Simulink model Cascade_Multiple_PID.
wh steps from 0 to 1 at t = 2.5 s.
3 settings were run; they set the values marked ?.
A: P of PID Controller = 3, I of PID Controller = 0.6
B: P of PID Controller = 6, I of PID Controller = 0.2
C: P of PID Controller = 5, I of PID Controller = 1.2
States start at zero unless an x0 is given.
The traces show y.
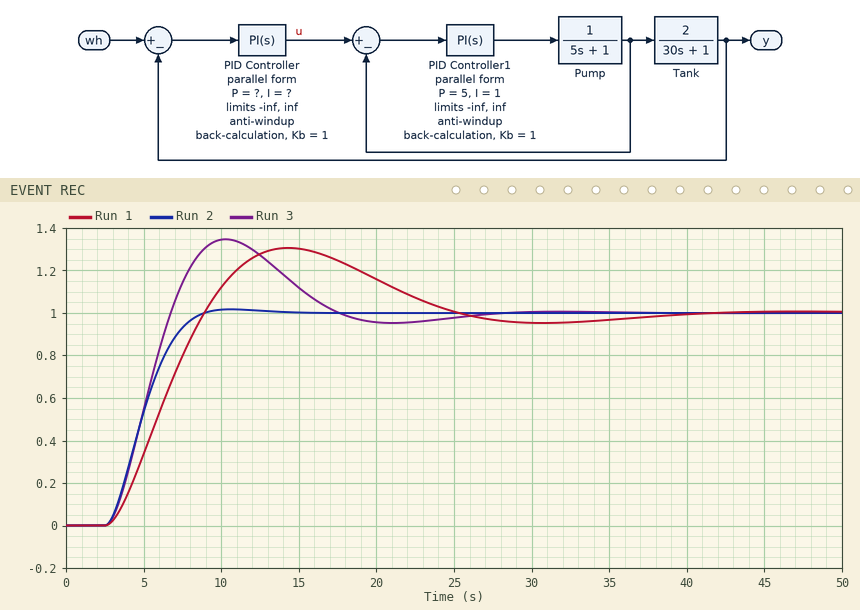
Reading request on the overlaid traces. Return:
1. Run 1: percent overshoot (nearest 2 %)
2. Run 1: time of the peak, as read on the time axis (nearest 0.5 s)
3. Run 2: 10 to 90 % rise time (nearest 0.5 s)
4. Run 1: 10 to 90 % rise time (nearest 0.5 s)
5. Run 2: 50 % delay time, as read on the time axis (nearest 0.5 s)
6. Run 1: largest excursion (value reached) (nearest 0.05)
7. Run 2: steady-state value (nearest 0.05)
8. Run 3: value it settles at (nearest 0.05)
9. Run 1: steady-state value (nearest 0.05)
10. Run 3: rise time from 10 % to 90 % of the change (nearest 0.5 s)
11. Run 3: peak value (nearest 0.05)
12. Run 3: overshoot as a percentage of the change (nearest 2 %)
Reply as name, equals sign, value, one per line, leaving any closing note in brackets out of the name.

Run 1: percent overshoot = 30 %
Run 1: time of the peak, as read on the time axis = 14.5 s
Run 2: 10 to 90 % rise time = 4.0 s
Run 1: 10 to 90 % rise time = 4.5 s
Run 2: 50 % delay time, as read on the time axis = 5.0 s
Run 1: largest excursion (value reached) = 1.30
Run 2: steady-state value = 1.00
Run 3: value it settles at = 1.00
Run 1: steady-state value = 1.00
Run 3: rise time from 10 % to 90 % of the change = 3.0 s
Run 3: peak value = 1.35
Run 3: overshoot as a percentage of the change = 34 %
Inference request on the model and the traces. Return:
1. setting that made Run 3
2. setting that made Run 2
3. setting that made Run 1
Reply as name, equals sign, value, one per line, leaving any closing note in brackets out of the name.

setting that made Run 3 = C
setting that made Run 2 = B
setting that made Run 1 = A
